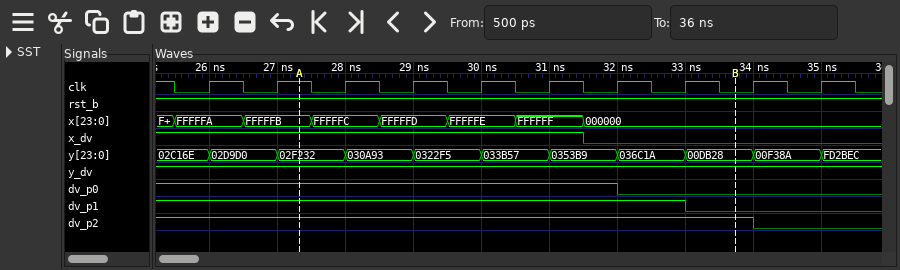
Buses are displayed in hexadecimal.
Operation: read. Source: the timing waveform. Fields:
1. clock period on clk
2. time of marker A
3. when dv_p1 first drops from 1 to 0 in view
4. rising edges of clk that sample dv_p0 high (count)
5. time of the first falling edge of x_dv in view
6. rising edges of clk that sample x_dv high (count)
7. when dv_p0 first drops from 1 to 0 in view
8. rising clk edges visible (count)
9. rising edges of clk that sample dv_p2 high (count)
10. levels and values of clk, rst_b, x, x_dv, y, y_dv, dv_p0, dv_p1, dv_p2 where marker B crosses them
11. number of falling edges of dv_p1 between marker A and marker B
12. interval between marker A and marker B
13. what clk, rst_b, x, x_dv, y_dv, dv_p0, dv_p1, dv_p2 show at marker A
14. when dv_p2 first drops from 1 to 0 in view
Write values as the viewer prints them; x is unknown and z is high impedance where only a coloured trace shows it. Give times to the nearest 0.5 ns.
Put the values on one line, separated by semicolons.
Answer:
1 ns; 27.5 ns; 33 ns; 7; 31.5 ns; 6; 32 ns; 10; 9; clk=0, rst_b=1, x=000000, x_dv=0, y=00DB28, y_dv=1, dv_p0=0, dv_p1=0, dv_p2=1; 1; 6.5 ns; clk=1, rst_b=1, x=FFFFFB, x_dv=1, y_dv=1, dv_p0=1, dv_p1=1, dv_p2=1; 34 ns
